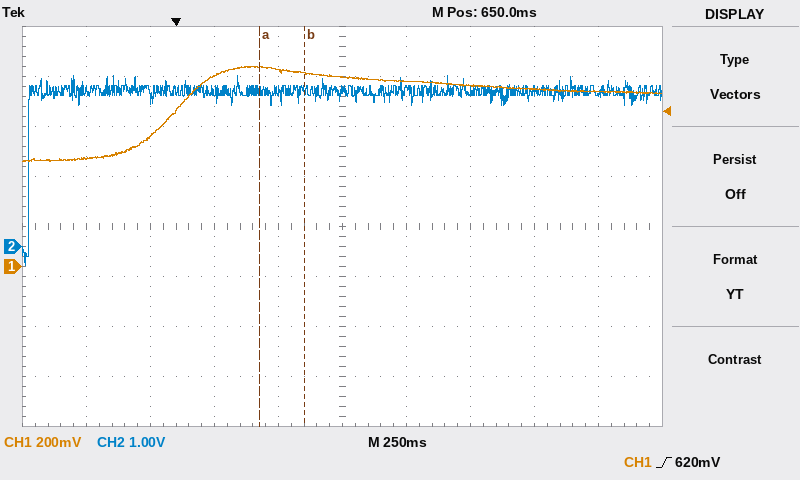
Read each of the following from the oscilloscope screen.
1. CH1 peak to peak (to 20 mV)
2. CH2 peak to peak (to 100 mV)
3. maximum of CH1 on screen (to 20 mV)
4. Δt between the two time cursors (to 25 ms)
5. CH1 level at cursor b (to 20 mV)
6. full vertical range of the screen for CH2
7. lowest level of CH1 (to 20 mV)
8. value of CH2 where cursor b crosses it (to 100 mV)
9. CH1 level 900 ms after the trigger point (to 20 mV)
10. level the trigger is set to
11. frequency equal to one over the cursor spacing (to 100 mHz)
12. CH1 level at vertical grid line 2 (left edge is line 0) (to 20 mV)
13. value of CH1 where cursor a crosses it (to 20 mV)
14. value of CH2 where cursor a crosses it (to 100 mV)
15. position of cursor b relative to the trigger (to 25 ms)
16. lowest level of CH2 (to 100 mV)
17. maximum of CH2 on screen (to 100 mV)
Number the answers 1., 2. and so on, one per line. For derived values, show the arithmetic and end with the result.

1. 800 mV − (420 mV) = 380 mV
2. 3.4 V − (-400 mV) = 3.8 V
3. 800 mV
4. 175 ms
5. 780 mV
6. 8 V
7. 420 mV
8. 3.1 V
9. 740 mV
10. 620 mV
11. 1 / 175 ms ≈ 5.7 Hz
12. 520 mV
13. 800 mV
14. 3.1 V
15. +500 ms
16. -400 mV
17. 3.4 V
